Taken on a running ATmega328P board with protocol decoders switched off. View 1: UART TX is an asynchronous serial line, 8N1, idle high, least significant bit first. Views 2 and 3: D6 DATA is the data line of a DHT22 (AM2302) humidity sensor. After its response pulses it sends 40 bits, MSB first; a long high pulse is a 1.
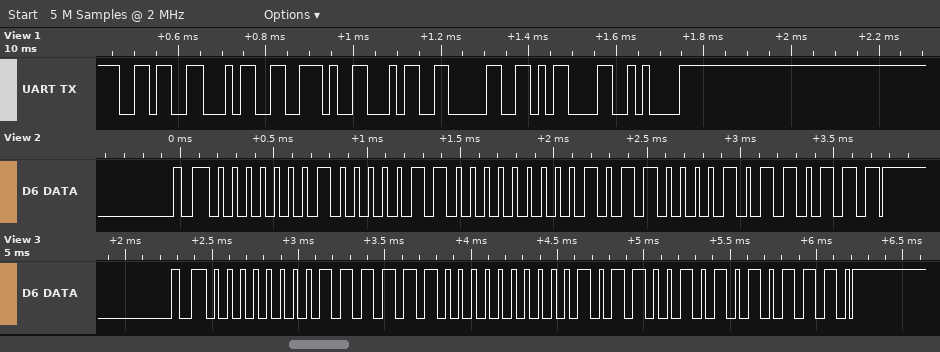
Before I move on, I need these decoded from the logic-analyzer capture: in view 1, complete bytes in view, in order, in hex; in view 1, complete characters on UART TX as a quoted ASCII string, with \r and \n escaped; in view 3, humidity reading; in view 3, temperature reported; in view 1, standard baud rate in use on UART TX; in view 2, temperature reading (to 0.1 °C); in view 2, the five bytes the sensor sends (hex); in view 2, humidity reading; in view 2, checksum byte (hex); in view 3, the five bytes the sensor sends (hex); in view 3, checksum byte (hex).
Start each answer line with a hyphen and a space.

- 36 34 2E 34 30 0D 0A
- "64.40\r\n"
- 25.2 %
- 17.8 °C
- 57600 baud
- 17.6 °C
- 01 06 00 B0 B7
- 26.2 %
- 0xB7
- 00 FC 00 B2 AE
- 0xAE
